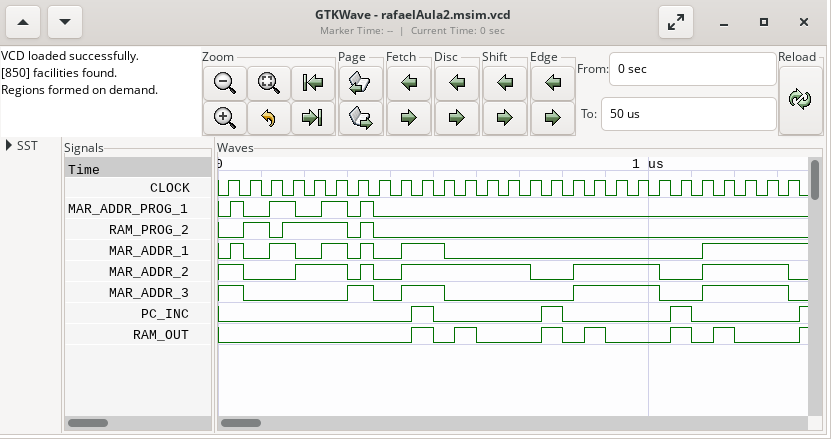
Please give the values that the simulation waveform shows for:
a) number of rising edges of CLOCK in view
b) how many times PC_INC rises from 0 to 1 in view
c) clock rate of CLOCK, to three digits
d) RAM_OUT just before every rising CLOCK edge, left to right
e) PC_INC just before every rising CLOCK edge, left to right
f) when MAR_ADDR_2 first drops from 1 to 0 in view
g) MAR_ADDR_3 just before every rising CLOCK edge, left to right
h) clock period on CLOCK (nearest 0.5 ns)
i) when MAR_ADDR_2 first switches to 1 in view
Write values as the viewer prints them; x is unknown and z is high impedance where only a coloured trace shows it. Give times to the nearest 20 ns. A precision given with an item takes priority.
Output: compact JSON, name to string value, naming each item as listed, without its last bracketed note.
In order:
{"number of rising edges of CLOCK in view": "27", "how many times PC_INC rises from 0 to 1 in view": "4", "clock rate of CLOCK, to three digits": "20.0 MHz", "RAM_OUT just before every rising CLOCK edge, left to right": "0 0 0 0 0 0 0 0 0 1 0 1 0 0 0 1 0 1 0 0 0 1 0 1 0 0 0", "PC_INC just before every rising CLOCK edge, left to right": "0 0 0 0 0 0 0 0 0 1 0 0 0 0 0 1 0 0 0 0 0 1 0 0 0 0 0", "when MAR_ADDR_2 first drops from 1 to 0 in view": "60 ns", "MAR_ADDR_3 just before every rising CLOCK edge, left to right": "1 0 0 0 0 0 1 0 0 1 1 0 0 0 0 0 0 1 1 1 1 0 0 1 1 1 1", "clock period on CLOCK": "50 ns", "when MAR_ADDR_2 first switches to 1 in view": "180 ns"}
